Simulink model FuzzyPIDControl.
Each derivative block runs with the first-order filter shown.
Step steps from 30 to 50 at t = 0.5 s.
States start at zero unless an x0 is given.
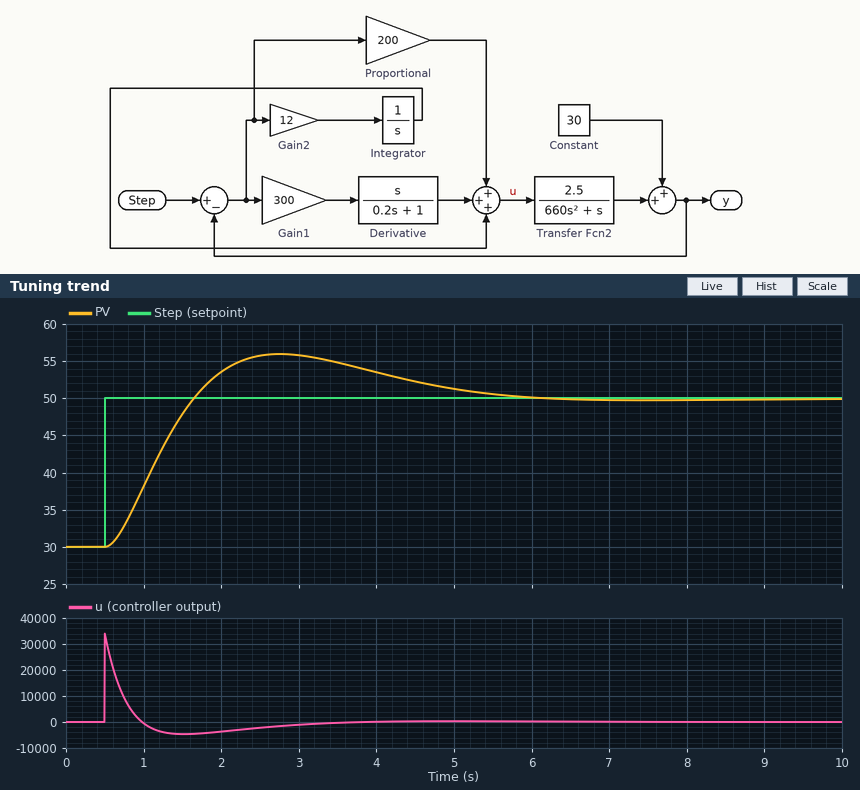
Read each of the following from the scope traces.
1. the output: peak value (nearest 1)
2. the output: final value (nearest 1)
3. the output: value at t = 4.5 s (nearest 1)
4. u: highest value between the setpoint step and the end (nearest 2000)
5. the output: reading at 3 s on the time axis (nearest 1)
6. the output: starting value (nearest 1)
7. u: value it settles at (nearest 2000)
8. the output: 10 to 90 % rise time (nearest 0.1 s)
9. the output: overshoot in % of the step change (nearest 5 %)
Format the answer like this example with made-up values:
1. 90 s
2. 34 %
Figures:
1. 56
2. 50
3. 52
4. 34000
5. 56
6. 30
7. 0
8. 0.8 s
9. 30 %
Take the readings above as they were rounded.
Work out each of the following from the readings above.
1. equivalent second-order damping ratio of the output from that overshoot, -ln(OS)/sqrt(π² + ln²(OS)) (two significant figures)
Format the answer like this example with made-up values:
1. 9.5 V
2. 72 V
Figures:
1. 0.36
